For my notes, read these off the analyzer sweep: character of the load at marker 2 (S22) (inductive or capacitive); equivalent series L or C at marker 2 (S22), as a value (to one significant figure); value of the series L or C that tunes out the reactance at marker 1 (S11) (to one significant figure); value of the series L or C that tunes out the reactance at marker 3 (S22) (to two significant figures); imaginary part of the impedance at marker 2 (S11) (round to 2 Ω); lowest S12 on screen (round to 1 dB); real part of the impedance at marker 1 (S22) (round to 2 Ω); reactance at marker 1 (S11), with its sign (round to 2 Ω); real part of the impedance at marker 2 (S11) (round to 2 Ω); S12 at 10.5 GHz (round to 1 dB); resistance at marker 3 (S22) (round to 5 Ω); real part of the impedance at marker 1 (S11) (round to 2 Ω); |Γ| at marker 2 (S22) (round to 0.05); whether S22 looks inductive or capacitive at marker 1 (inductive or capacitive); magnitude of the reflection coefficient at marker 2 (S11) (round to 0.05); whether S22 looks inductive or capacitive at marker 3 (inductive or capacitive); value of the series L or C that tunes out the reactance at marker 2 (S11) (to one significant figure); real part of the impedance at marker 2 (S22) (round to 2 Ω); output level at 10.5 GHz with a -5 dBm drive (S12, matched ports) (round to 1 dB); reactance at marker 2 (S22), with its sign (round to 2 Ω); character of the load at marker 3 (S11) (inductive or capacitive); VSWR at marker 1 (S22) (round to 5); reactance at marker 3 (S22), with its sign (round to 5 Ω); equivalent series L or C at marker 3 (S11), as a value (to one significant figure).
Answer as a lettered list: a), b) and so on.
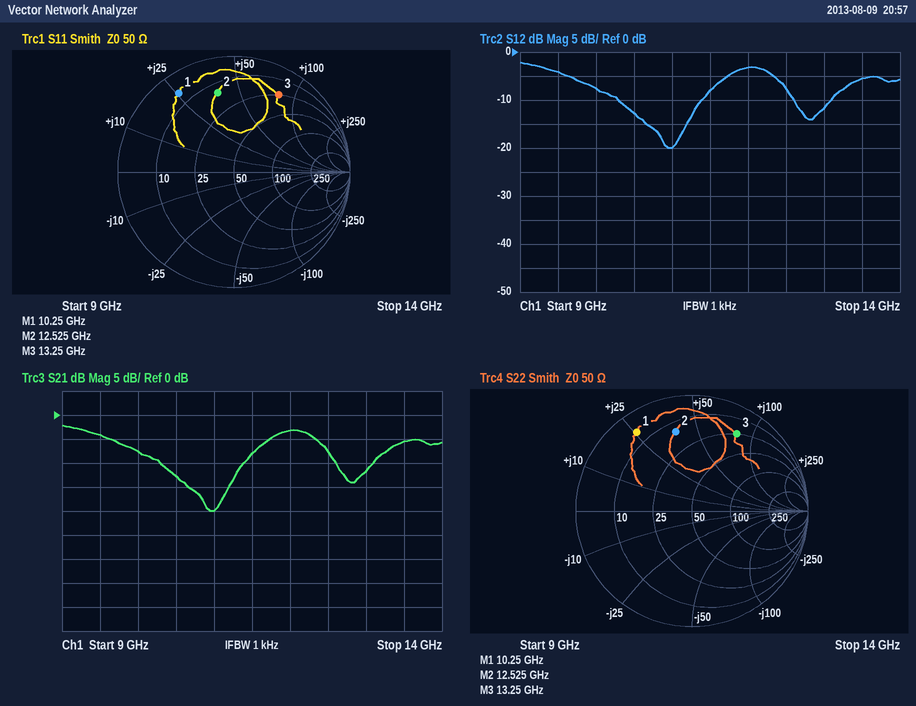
a) inductive
b) 500 pH
c) 600 fF
d) 150 fF
e) +38 Ω
f) -20 dB
g) 6 Ω
h) +26 Ω
i) 14 Ω
j) -13 dB
k) 25 Ω
l) 6 Ω
m) 0.70
n) inductive
o) 0.70
p) inductive
q) 300 fF
r) 14 Ω
s) -18 dBm
t) +38 Ω
u) inductive
v) 10
w) +80 Ω
x) 1.0 nH
